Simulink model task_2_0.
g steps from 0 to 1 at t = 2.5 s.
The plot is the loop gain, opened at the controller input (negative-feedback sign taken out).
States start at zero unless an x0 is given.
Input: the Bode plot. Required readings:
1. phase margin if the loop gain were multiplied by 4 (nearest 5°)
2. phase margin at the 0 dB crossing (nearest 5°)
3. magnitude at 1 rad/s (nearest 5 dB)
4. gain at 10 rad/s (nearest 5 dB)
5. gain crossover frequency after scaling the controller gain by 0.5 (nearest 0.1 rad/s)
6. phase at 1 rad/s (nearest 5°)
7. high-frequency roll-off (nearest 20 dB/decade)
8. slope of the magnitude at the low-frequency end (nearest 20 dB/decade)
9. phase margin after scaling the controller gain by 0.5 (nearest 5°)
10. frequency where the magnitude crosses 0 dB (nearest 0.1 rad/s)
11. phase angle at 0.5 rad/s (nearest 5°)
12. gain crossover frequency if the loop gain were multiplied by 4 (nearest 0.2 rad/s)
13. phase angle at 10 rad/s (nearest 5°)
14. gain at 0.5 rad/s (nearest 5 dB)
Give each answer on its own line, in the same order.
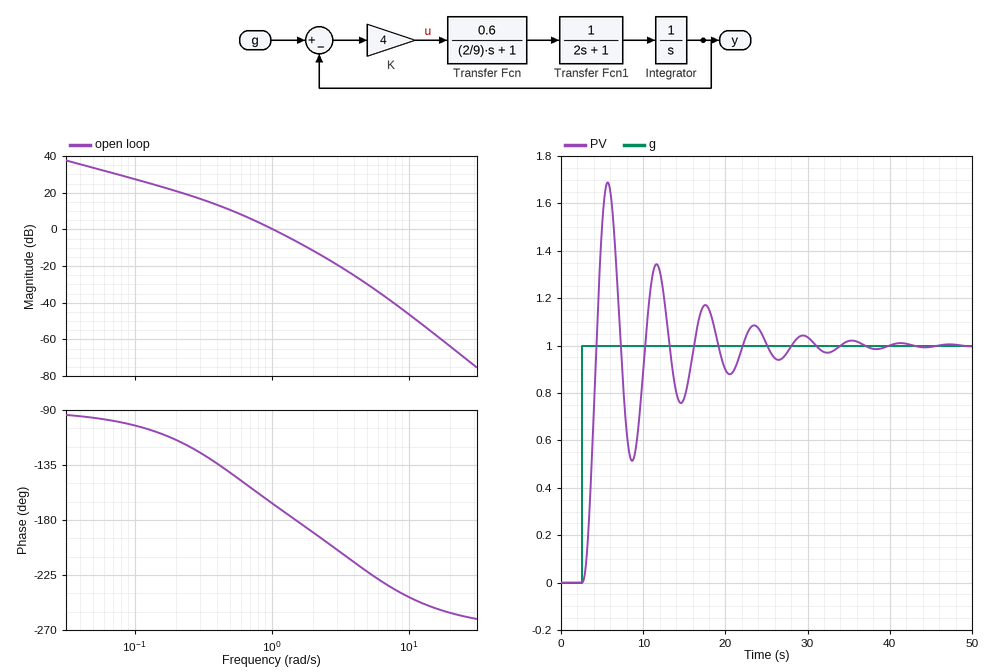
-10°
15°
0 dB
-45 dB
0.7 rad/s
-165°
-60 dB/decade
-20 dB/decade
25°
1.0 rad/s
-140°
2.0 rad/s
-245°
10 dB
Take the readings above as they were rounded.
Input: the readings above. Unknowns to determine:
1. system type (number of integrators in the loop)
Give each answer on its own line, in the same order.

1
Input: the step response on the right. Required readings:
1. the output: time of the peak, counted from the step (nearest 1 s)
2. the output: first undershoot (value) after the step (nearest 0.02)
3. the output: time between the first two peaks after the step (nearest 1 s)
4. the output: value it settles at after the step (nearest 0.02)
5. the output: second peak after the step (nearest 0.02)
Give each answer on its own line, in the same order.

3 s
0.52
6 s
1.00
1.34
